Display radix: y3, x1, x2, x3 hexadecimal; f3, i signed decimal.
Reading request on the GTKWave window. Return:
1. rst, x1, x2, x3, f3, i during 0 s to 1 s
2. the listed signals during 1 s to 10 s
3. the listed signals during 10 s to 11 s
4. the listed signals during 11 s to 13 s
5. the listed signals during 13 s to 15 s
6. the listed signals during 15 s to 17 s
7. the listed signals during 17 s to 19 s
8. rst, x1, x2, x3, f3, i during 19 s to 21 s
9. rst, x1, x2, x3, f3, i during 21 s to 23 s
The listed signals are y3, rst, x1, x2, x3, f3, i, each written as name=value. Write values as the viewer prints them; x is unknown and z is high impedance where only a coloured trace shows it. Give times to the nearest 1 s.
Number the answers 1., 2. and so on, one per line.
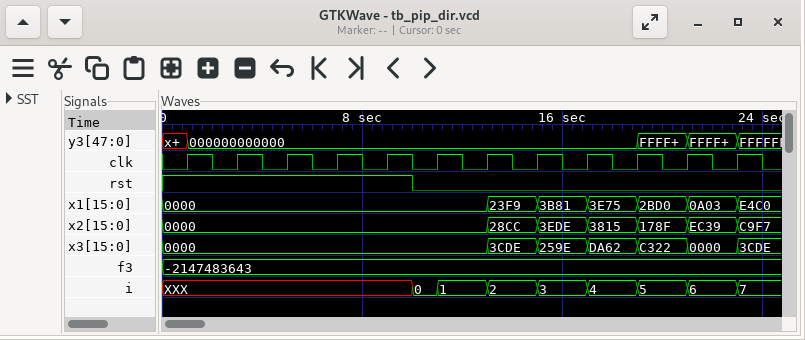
1. rst=1, x1=0000, x2=0000, x3=0000, f3=-2147483643, i=XXX
2. y3=000000000000, rst=1, x1=0000, x2=0000, x3=0000, f3=-2147483643, i=XXX
3. y3=000000000000, rst=0, x1=0000, x2=0000, x3=0000, f3=-2147483643, i=0
4. y3=000000000000, rst=0, x1=0000, x2=0000, x3=0000, f3=-2147483643, i=1
5. y3=000000000000, rst=0, x1=23F9, x2=28CC, x3=3CDE, f3=-2147483643, i=2
6. y3=000000000000, rst=0, x1=3B81, x2=3EDE, x3=259E, f3=-2147483643, i=3
7. y3=000000000000, rst=0, x1=3E75, x2=3815, x3=DA62, f3=-2147483643, i=4
8. rst=0, x1=2BD0, x2=178F, x3=C322, f3=-2147483643, i=5
9. rst=0, x1=0A03, x2=EC39, x3=0000, f3=-2147483643, i=6
